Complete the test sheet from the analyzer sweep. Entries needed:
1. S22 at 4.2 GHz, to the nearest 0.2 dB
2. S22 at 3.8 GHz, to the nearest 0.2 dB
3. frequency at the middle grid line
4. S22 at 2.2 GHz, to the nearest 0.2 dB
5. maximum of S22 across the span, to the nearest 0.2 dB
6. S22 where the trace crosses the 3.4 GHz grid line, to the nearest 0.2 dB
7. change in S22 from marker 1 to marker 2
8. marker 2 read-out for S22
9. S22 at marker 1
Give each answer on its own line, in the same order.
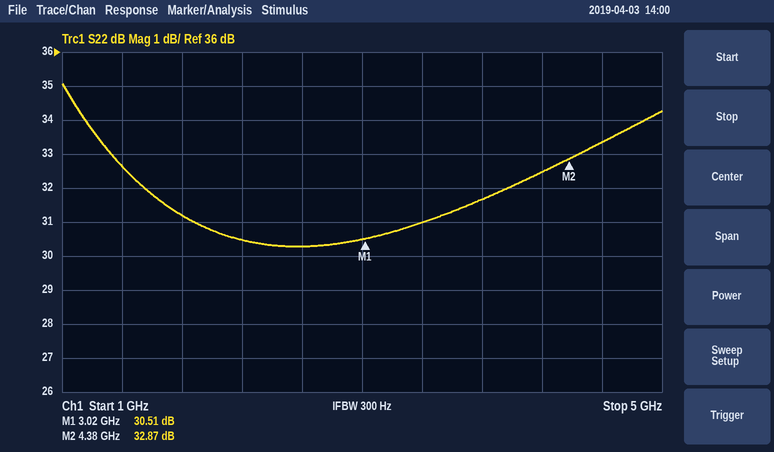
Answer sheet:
32.4 dB
31.6 dB
3 GHz
30.4 dB
35.0 dB
31.0 dB
2.36 dB
32.87 dB
30.51 dB
